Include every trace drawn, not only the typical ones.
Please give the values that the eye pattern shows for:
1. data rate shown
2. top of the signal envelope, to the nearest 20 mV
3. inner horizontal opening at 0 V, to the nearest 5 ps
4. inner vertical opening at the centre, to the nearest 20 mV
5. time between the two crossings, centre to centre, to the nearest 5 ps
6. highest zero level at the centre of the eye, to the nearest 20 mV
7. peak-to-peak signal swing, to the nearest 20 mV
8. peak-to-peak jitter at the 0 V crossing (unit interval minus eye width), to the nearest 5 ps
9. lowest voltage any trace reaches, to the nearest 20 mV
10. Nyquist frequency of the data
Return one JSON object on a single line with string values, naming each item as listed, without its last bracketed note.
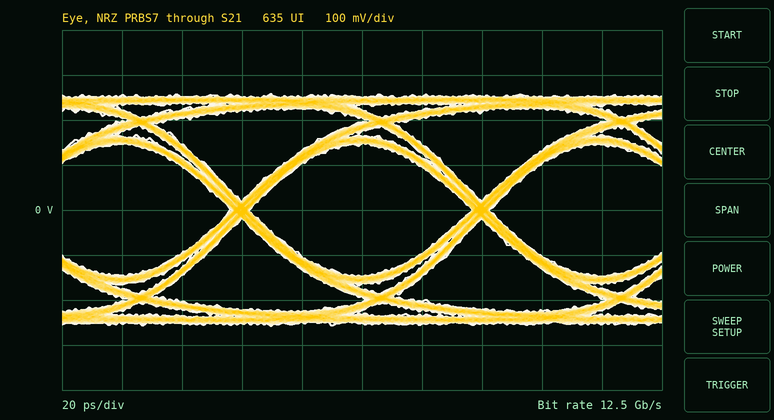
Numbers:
{"data rate shown": "12.5 Gb/s", "top of the signal envelope, to the nearest 20 mV": "260 mV", "inner horizontal opening at 0 V, to the nearest 5 ps": "75 ps", "inner vertical opening at the centre, to the nearest 20 mV": "300 mV", "time between the two crossings, centre to centre, to the nearest 5 ps": "80 ps", "highest zero level at the centre of the eye, to the nearest 20 mV": "-140 mV", "peak-to-peak signal swing, to the nearest 20 mV": "520 mV", "peak-to-peak jitter at the 0 V crossing (unit interval minus eye width), to the nearest 5 ps": "5 ps", "lowest voltage any trace reaches, to the nearest 20 mV": "-260 mV", "Nyquist frequency of the data": "6.25 GHz"}
